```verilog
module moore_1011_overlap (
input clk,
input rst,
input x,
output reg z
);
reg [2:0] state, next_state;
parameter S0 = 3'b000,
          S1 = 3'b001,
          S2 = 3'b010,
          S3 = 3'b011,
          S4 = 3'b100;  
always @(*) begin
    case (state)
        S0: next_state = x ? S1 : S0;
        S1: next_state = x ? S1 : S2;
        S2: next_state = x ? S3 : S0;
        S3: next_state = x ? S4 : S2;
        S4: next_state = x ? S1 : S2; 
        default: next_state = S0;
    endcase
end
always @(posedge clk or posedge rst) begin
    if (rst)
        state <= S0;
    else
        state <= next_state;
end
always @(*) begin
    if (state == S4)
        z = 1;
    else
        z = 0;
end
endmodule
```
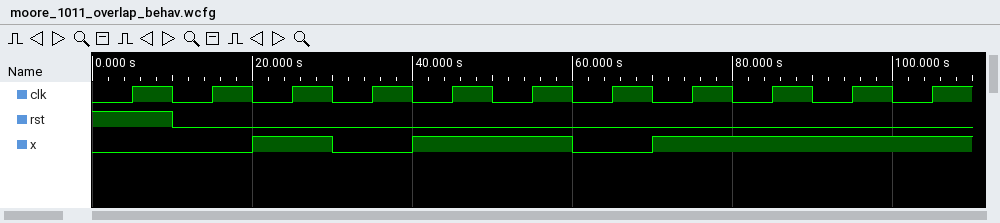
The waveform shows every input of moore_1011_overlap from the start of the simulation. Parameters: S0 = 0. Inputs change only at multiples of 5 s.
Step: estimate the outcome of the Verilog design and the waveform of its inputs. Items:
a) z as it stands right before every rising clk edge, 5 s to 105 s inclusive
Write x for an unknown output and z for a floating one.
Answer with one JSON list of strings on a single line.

["0 0 0 0 0 0 1 0 0 1 0"]
